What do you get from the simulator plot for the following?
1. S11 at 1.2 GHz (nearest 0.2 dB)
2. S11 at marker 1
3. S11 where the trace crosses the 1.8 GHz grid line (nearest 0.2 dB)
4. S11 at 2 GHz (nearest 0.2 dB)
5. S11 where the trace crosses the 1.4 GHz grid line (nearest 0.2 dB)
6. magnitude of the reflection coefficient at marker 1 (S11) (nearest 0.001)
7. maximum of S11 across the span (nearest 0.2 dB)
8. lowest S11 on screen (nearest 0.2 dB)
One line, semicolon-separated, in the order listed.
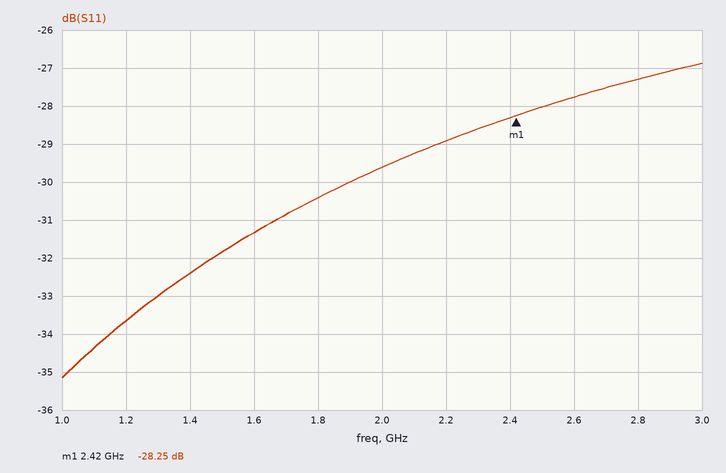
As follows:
-33.6 dB; -28.25 dB; -30.4 dB; -29.6 dB; -32.4 dB; 0.039; -26.8 dB; -35.2 dB
